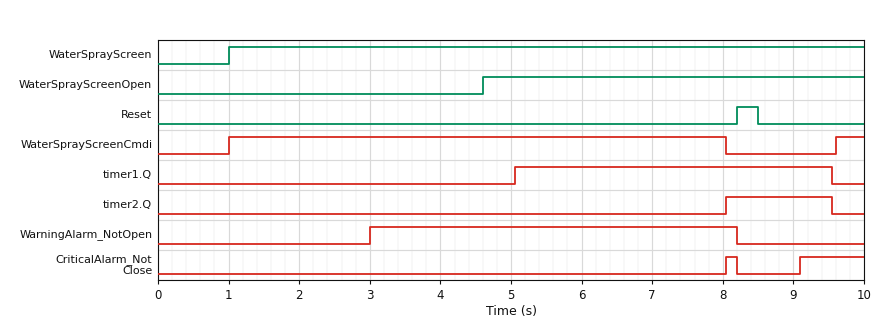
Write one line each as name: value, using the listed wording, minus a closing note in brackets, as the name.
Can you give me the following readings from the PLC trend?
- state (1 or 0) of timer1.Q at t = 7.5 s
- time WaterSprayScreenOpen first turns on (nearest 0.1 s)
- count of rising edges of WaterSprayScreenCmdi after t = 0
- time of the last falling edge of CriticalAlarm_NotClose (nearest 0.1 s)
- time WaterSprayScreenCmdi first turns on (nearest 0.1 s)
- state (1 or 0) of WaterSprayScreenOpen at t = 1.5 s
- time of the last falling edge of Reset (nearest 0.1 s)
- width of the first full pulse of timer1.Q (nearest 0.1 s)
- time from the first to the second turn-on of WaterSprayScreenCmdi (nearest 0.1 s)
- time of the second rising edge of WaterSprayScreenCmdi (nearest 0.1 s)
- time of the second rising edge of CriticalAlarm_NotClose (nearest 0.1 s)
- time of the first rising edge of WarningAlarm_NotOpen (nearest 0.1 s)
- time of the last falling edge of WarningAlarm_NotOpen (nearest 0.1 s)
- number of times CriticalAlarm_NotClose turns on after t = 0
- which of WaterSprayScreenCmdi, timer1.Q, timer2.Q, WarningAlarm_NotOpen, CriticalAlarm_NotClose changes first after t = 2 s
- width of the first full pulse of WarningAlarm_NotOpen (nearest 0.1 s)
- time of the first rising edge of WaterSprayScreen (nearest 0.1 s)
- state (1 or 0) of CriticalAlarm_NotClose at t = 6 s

state (1 or 0) of timer1.Q at t = 7.5 s: 1
time WaterSprayScreenOpen first turns on: 4.6 s
count of rising edges of WaterSprayScreenCmdi after t = 0: 2
time of the last falling edge of CriticalAlarm_NotClose: 8.2 s
time WaterSprayScreenCmdi first turns on: 1.0 s
state (1 or 0) of WaterSprayScreenOpen at t = 1.5 s: 0
time of the last falling edge of Reset: 8.5 s
width of the first full pulse of timer1.Q: 4.5 s
time from the first to the second turn-on of WaterSprayScreenCmdi: 8.6 s
time of the second rising edge of WaterSprayScreenCmdi: 9.6 s
time of the second rising edge of CriticalAlarm_NotClose: 9.1 s
time of the first rising edge of WarningAlarm_NotOpen: 3.0 s
time of the last falling edge of WarningAlarm_NotOpen: 8.2 s
number of times CriticalAlarm_NotClose turns on after t = 0: 2
which of WaterSprayScreenCmdi, timer1.Q, timer2.Q, WarningAlarm_NotOpen, CriticalAlarm_NotClose changes first after t = 2 s: WarningAlarm_NotOpen
width of the first full pulse of WarningAlarm_NotOpen: 5.2 s
time of the first rising edge of WaterSprayScreen: 1.0 s
state (1 or 0) of CriticalAlarm_NotClose at t = 6 s: 0
